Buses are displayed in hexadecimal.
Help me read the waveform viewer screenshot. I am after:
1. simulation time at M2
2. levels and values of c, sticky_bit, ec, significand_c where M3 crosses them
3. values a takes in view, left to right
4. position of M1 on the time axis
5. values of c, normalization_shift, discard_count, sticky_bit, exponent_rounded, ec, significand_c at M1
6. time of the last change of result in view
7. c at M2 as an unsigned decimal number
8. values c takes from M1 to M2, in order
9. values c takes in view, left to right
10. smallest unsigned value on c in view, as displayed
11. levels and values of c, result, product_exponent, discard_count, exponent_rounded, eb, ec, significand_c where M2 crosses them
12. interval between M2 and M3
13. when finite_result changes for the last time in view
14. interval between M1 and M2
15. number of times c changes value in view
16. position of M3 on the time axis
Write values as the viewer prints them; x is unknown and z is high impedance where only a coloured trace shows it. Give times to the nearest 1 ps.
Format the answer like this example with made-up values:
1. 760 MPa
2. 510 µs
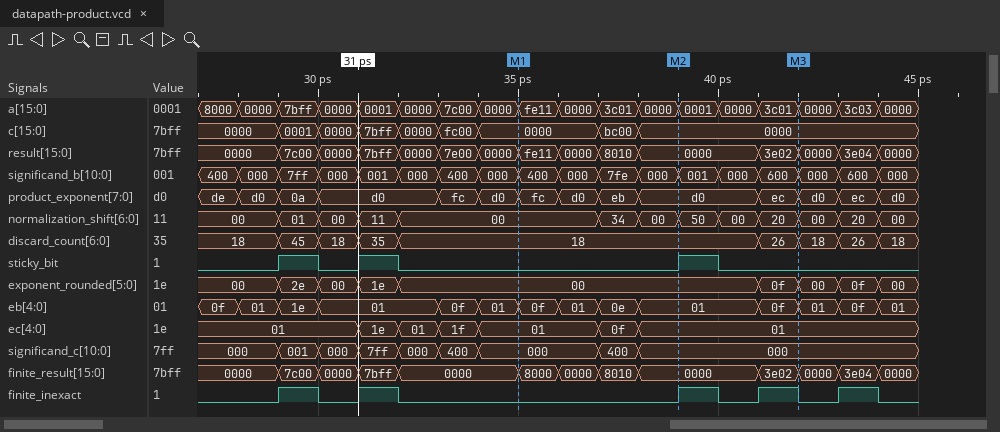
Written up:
1. 39 ps
2. c=0000, sticky_bit=0, ec=01, significand_c=000
3. 8000, 0000, 7bff, 0000, 0001, 0000, 7c00, 0000, fe11, 0000, 3c01, 0000, 0001, 0000, 3c01, 0000, 3c03, 0000
4. 35 ps
5. c=0000, normalization_shift=00, discard_count=18, sticky_bit=0, exponent_rounded=00, ec=01, significand_c=000
6. 44 ps
7. 0
8. 0000, bc00, 0000
9. 0000, 0001, 0000, 7bff, 0000, fc00, 0000, bc00, 0000
10. 0000
11. c=0000, result=0000, product_exponent=d0, discard_count=18, exponent_rounded=00, eb=01, ec=01, significand_c=000
12. 3 ps
13. 44 ps
14. 4 ps
15. 8
16. 42 ps
